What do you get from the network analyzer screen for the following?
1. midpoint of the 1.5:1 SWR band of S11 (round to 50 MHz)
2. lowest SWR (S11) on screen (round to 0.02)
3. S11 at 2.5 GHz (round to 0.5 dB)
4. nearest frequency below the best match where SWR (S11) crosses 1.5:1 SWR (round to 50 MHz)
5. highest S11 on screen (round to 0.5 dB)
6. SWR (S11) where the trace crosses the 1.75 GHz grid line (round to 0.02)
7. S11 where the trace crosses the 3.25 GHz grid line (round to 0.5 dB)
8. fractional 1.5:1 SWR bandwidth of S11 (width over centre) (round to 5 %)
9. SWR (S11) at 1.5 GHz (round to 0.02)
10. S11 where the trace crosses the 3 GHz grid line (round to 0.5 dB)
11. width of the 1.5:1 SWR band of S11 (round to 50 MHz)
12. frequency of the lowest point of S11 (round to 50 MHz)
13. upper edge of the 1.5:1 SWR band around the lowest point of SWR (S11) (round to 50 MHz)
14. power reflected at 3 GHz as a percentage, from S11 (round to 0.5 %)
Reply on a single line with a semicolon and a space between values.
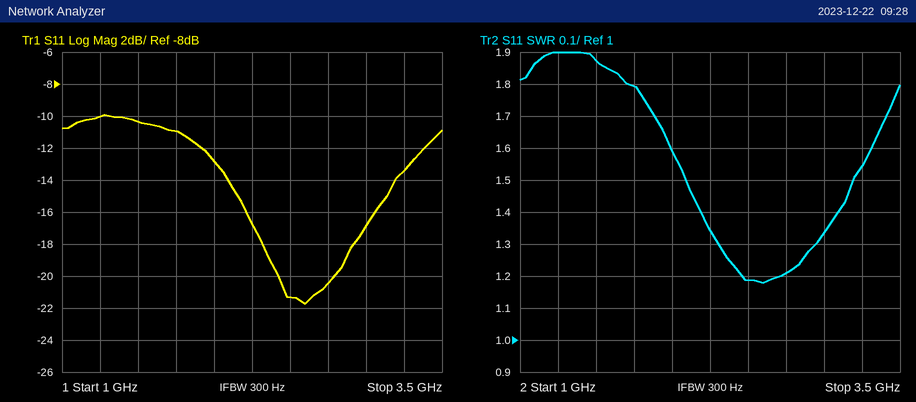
2.65 GHz; 1.18; -21.5 dB; 2.10 GHz; -10.0 dB; 1.80; -13.5 dB; 40 %; 1.88; -17.0 dB; 1.10 GHz; 2.60 GHz; 3.20 GHz; 2.0 %
